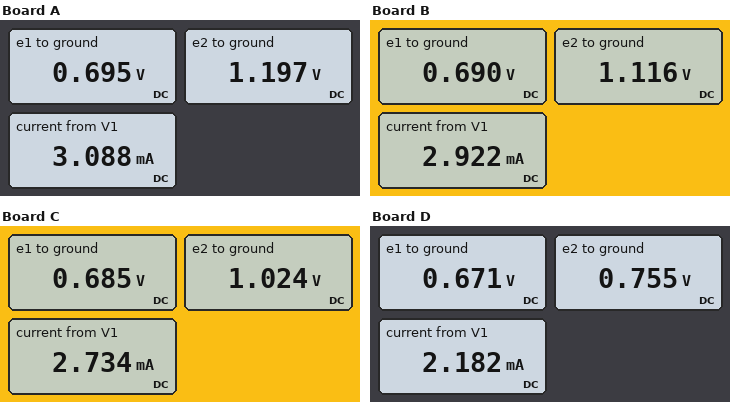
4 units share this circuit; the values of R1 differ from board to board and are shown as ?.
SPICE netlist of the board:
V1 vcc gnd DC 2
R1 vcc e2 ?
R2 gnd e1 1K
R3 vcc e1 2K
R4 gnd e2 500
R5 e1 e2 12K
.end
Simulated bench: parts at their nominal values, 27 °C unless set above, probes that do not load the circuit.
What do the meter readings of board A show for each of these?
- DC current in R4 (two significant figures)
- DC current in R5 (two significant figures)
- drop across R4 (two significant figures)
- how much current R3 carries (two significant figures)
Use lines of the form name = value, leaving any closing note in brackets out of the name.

DC current in R4 = 2.4 mA
DC current in R5 = 42 µA
drop across R4 = 1.2 V
how much current R3 carries = 650 µA
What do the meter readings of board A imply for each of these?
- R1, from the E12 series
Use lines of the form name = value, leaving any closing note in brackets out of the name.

R1, from the E12 series = 330 Ω
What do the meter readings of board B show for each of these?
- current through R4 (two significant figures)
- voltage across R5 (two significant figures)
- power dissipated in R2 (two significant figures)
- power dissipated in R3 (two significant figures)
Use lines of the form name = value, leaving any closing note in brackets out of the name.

current through R4 = 2.2 mA
voltage across R5 = 430 mV
power dissipated in R2 = 480 µW
power dissipated in R3 = 860 µW
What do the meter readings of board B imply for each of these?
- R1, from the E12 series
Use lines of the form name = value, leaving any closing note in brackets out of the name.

R1, from the E12 series = 390 Ω
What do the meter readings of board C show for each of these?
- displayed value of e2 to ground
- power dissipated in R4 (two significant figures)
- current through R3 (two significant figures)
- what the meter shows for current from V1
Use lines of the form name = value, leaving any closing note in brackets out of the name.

displayed value of e2 to ground = 1.024 V
power dissipated in R4 = 2.1 mW
current through R3 = 660 µA
what the meter shows for current from V1 = 2.734 mA
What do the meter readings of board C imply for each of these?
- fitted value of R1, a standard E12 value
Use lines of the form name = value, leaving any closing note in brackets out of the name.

fitted value of R1, a standard E12 value = 470 Ω
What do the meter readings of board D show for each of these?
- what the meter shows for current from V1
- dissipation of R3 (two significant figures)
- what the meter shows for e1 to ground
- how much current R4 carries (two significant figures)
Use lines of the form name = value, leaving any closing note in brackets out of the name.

what the meter shows for current from V1 = 2.182 mA
dissipation of R3 = 880 µW
what the meter shows for e1 to ground = 0.671 V
how much current R4 carries = 1.5 mA
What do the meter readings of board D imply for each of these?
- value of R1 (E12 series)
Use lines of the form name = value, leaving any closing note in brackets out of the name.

value of R1 = 820 Ω
